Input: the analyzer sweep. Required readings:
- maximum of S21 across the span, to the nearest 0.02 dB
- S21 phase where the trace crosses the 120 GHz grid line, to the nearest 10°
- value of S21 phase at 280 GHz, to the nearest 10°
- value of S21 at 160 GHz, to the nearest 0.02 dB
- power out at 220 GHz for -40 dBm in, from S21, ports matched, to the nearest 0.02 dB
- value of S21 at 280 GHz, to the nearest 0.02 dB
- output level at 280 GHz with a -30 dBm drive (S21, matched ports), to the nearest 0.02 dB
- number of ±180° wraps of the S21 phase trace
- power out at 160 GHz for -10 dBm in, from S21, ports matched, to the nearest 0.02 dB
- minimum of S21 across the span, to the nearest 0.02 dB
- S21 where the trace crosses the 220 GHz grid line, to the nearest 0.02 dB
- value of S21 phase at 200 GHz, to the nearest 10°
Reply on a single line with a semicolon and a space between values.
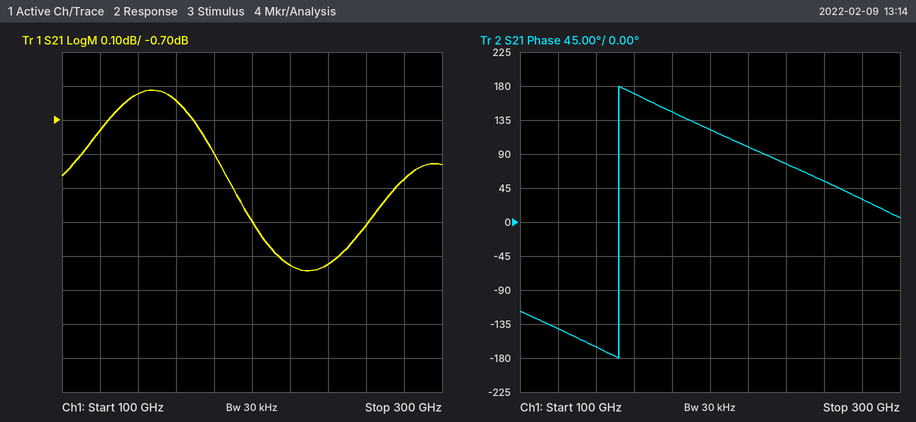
-0.62 dB; -140°; 30°; -0.64 dB; -41.12 dBm; -0.88 dB; -30.88 dBm; 1; -10.64 dBm; -1.14 dB; -1.12 dB; 120°
